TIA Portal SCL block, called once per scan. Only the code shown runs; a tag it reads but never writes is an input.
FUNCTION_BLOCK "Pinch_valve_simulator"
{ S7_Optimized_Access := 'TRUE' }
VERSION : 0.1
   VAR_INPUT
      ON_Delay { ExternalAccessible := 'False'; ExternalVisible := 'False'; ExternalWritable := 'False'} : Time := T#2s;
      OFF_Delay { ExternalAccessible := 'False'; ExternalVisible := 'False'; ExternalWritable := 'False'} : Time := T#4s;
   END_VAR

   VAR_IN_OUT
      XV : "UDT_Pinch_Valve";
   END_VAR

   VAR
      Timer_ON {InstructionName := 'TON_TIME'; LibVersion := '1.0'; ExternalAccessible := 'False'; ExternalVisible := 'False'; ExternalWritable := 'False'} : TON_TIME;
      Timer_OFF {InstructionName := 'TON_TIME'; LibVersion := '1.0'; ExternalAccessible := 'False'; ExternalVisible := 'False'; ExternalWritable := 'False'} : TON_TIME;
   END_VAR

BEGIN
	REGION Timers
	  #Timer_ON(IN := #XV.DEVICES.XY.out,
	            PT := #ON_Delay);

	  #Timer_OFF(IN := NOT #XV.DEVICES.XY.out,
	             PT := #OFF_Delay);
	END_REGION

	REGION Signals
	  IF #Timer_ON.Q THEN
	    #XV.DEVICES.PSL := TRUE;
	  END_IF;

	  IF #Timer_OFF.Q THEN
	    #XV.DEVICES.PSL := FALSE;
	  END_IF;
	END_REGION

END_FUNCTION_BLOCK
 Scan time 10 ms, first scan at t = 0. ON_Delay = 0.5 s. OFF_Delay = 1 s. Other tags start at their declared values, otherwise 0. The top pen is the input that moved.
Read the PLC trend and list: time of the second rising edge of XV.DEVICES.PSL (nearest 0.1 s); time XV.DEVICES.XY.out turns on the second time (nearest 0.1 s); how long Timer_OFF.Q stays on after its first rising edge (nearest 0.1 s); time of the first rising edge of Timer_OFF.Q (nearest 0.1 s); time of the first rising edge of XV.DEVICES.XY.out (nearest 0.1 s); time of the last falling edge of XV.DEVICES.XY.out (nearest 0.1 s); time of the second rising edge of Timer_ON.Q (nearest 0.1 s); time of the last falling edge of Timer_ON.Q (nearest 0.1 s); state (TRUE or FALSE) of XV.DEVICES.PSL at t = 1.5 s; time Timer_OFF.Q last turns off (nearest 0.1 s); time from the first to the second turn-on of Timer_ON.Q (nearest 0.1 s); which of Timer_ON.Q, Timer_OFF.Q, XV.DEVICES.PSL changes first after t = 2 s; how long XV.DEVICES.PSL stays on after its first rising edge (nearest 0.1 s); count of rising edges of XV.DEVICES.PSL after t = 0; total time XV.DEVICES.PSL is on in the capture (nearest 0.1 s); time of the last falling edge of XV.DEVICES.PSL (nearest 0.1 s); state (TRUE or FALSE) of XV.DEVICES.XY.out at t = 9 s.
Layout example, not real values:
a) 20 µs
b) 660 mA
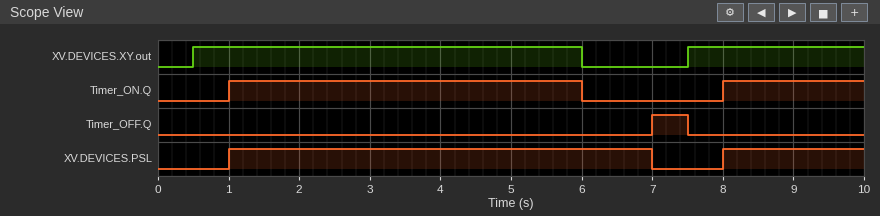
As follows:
a) 8.0 s
b) 7.5 s
c) 0.5 s
d) 7.0 s
e) 0.5 s
f) 6.0 s
g) 8.0 s
h) 6.0 s
i) TRUE
j) 7.5 s
k) 7.0 s
l) Timer_ON.Q
m) 6.0 s
n) 2
o) 8.0 s
p) 7.0 s
q) TRUE
